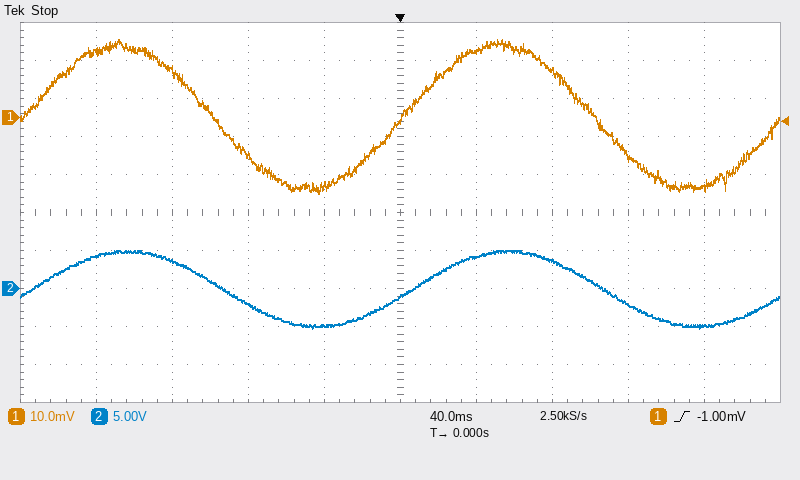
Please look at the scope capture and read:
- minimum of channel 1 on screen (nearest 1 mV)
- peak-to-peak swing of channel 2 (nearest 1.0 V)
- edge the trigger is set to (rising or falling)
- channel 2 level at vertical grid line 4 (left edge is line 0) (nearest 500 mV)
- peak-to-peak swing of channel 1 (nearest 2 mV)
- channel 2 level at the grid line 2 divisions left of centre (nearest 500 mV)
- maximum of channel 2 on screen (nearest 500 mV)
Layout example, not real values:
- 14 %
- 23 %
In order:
- -20 mV
- 10.0 V
- rising
- -5.0 V
- 40 mV
- -2.0 V
- 5.0 V
